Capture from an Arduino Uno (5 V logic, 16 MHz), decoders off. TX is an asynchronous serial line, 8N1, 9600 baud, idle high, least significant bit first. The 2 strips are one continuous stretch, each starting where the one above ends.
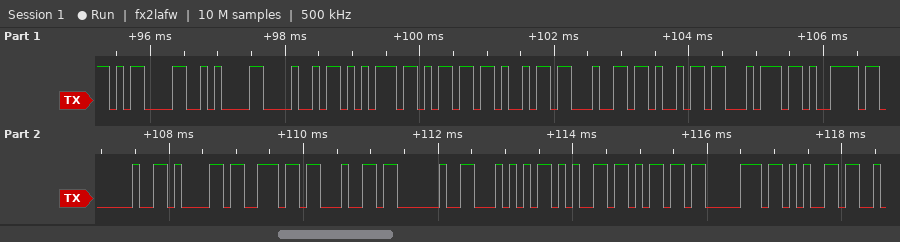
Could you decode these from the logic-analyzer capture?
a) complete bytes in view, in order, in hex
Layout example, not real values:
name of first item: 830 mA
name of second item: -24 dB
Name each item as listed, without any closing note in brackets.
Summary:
complete bytes in view, in order, in hex: 0x0D 0x0A 0x48 0x75 0x6D 0x69 0x64 0x69 0x74 0x79 0x20 0x61 0x6E 0x64 0x20 0x54 0x65 0x6D 0x70 0x65
